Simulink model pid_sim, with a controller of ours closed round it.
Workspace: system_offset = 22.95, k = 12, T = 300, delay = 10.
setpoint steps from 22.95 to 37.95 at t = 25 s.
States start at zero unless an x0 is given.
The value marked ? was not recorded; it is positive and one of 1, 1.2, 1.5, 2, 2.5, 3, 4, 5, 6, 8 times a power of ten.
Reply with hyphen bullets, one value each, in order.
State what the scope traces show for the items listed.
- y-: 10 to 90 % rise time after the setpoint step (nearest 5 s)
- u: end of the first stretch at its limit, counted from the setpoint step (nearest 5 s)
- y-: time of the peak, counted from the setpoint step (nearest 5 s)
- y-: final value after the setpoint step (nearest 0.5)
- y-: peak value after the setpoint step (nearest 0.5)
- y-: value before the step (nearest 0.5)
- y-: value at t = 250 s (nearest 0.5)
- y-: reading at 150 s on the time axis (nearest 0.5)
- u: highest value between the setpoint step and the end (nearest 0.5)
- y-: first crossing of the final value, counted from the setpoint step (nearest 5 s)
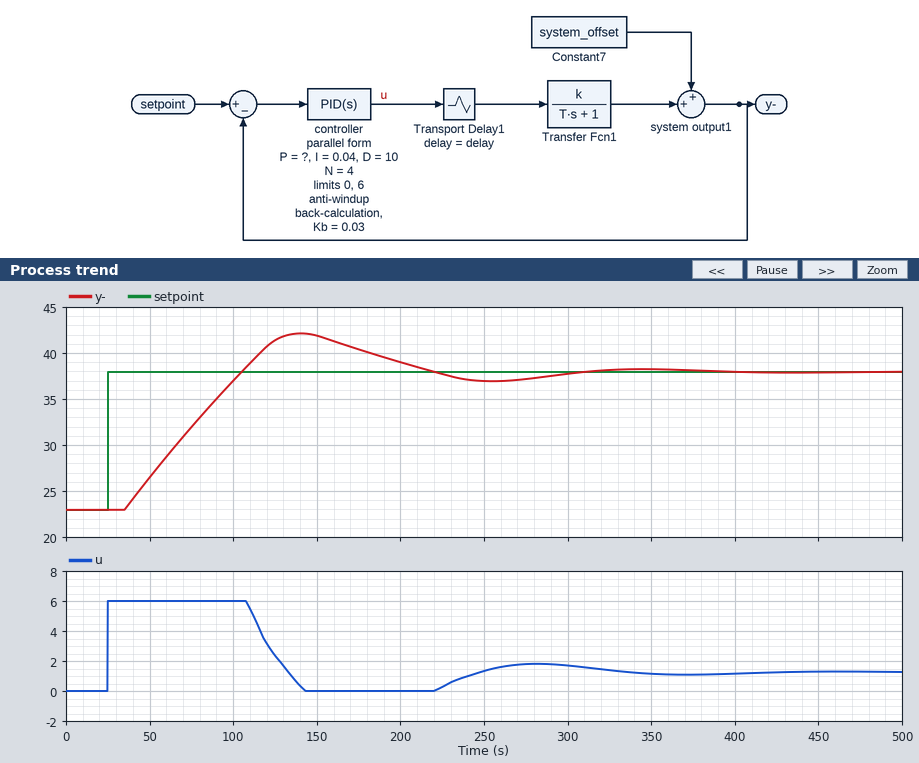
- 55 s
- 85 s
- 115 s
- 38.0
- 42.0
- 23.0
- 37.0
- 42.0
- 6.0
- 80 s
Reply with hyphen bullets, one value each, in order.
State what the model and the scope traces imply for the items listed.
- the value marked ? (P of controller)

- 1
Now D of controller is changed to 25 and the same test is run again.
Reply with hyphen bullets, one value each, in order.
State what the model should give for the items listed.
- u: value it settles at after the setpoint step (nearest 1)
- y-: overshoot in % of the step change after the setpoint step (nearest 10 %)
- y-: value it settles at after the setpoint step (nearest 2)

- 1
- 30 %
- 38
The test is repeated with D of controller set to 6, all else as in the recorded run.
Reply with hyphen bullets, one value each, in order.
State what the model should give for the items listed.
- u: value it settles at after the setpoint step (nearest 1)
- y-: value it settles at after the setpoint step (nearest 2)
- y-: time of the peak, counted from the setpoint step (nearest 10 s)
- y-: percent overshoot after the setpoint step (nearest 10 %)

- 1
- 38
- 110 s
- 30 %
